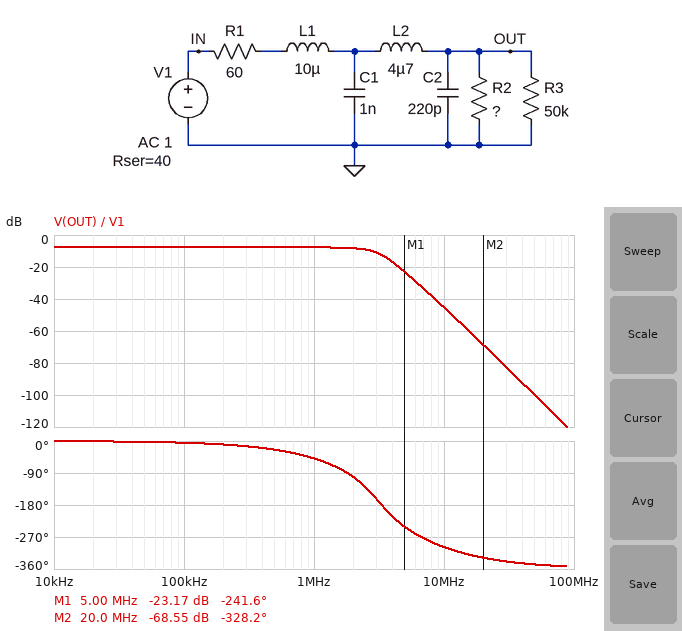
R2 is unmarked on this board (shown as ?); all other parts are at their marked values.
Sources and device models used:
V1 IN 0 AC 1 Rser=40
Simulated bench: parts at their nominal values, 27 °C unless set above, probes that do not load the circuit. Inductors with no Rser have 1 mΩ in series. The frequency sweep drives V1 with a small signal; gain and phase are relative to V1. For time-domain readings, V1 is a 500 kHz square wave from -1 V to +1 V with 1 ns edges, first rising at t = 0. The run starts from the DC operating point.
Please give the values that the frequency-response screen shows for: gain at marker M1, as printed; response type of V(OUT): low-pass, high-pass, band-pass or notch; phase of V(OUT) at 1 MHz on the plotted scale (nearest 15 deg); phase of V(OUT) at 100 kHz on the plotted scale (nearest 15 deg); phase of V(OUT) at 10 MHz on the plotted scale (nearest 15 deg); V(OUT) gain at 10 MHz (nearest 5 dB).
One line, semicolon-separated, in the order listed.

-23.17 dB; low-pass; -45 deg; 0 deg; -300 deg; -45 dB
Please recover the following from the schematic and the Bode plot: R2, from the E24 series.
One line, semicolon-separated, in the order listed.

75 Ω
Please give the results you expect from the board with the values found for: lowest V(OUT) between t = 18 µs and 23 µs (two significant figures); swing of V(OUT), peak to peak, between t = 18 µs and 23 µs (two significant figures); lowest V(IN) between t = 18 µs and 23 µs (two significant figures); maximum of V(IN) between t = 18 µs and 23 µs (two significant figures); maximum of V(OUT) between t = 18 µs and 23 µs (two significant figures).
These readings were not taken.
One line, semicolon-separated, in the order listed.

-480 mV; 960 mV; -1.2 V; 1.2 V; 480 mV
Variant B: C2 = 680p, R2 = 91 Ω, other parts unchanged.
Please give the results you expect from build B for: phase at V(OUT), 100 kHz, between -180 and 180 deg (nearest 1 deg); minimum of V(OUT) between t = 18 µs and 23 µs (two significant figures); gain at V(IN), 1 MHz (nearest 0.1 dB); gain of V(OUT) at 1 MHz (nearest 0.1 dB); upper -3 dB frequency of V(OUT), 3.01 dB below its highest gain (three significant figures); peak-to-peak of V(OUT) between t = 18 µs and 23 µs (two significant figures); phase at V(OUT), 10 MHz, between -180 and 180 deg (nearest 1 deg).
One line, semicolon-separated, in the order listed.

-6 deg; -520 mV; -2.3 dB; -6.8 dB; 3.42 MHz; 1.0 V; 25 deg
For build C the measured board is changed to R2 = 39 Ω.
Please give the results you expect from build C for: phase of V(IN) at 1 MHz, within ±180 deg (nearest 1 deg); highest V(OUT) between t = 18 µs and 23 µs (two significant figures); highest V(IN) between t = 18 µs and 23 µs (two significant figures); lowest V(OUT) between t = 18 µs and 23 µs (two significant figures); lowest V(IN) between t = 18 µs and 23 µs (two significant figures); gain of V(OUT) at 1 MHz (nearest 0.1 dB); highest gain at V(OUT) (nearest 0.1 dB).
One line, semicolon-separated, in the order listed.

8 deg; 330 mV; 1.3 V; -330 mV; -1.3 V; -11.6 dB; -10.7 dB
